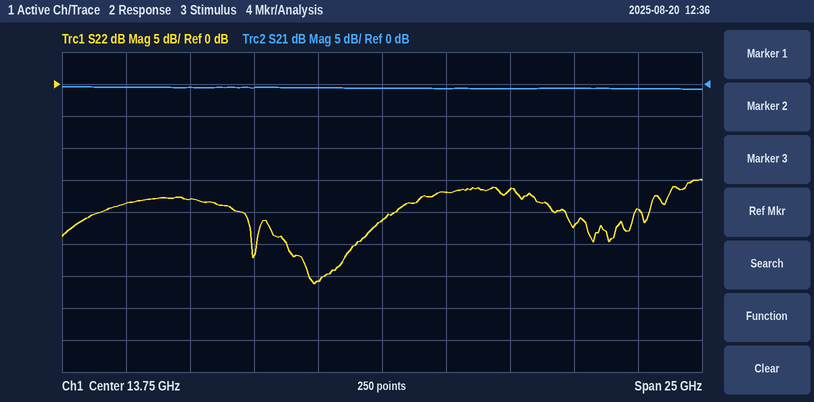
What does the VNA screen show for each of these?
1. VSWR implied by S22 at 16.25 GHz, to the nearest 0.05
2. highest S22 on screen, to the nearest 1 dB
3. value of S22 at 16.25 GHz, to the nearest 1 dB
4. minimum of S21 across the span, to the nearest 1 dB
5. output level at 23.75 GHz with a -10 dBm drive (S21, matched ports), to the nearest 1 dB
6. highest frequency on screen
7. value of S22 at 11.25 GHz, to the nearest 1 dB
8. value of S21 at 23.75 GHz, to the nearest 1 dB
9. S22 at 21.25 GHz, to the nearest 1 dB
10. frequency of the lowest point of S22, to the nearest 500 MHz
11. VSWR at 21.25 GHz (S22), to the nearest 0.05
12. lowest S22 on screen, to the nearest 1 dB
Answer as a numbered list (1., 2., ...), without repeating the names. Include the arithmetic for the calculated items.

1. |Γ| = 10^(-17/20) = 0.1413; VSWR = (1 + 0.1413)/(1 − 0.1413) ≈ 1.33, so 1.35 to the nearest 0.05
2. -15 dB
3. -17 dB
4. -1 dB
5. -10 dBm + (-1 dB) = -11 dBm
6. 26.25 GHz
7. -31 dB
8. -1 dB
9. -22 dB
10. 11.0 GHz
11. |Γ| = 10^(-22/20) = 0.0794; VSWR = (1 + 0.0794)/(1 − 0.0794) ≈ 1.17, so 1.15 to the nearest 0.05
12. -31 dB
